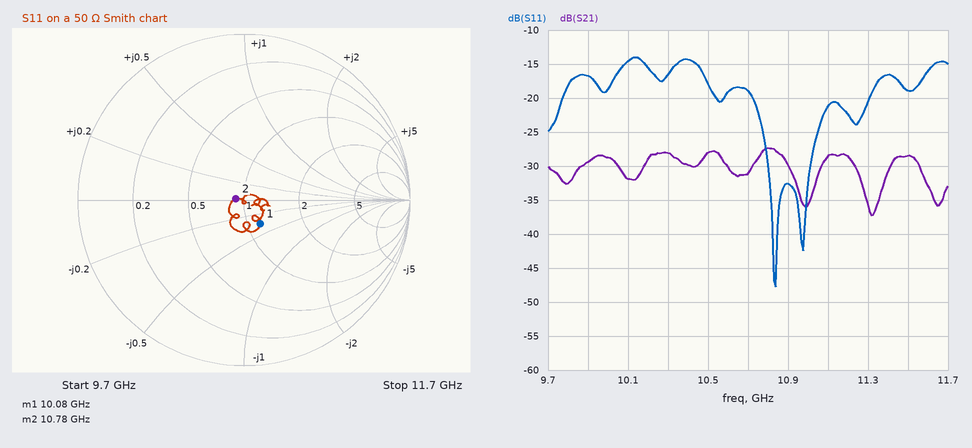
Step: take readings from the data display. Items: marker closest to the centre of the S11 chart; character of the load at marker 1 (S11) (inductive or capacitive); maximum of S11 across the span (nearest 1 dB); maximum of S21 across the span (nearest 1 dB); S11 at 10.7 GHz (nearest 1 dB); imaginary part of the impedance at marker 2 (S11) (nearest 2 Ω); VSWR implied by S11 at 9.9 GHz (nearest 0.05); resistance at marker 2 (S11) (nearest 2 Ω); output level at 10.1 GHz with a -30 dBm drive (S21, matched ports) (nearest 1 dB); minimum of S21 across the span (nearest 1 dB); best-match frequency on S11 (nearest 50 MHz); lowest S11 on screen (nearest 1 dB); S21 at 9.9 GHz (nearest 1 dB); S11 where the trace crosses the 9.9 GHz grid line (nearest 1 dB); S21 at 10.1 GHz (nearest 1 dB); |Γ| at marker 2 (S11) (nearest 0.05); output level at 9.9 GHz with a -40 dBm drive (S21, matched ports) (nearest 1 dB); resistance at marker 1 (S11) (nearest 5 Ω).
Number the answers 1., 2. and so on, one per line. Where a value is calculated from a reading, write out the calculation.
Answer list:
1. marker 2
2. capacitive
3. -14 dB
4. -27 dB
5. -19 dB
6. 0 Ω
7. |Γ| = 10^(-17/20) = 0.1413; VSWR = (1 + 0.1413)/(1 − 0.1413) ≈ 1.33, so 1.35 to the nearest 0.05
8. 46 Ω
9. -30 dBm + (-32 dB) = -62 dBm
10. -37 dB
11. 10.85 GHz
12. -48 dB
13. -29 dB
14. -17 dB
15. -32 dB
16. 0.05
17. -40 dBm + (-29 dB) = -69 dBm
18. 60 Ω
